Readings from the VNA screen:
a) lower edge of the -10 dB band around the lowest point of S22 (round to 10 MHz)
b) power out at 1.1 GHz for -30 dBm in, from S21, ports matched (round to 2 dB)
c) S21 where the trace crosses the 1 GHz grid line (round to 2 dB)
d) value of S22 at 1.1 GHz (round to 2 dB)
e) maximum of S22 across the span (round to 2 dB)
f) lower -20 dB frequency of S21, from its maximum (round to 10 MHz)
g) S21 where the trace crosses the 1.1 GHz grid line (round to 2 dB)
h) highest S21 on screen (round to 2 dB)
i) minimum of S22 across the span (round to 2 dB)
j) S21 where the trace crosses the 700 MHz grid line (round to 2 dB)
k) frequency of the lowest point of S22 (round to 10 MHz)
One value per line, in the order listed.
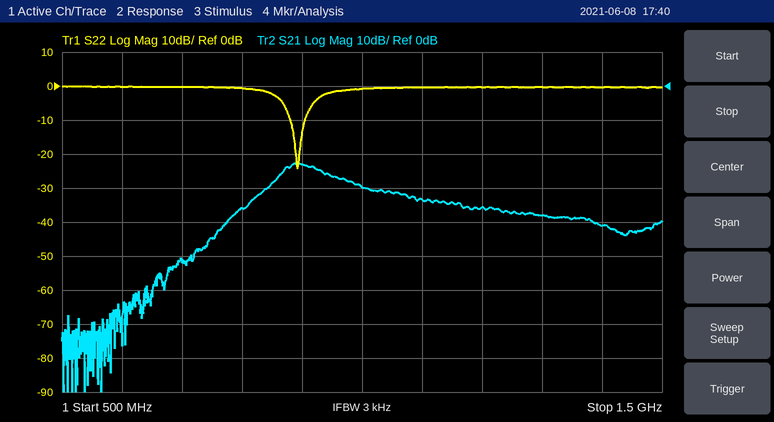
880 MHz
-64 dBm
-30 dB
0 dB
0 dB
760 MHz
-34 dB
-22 dB
-24 dB
-52 dB
890 MHz
